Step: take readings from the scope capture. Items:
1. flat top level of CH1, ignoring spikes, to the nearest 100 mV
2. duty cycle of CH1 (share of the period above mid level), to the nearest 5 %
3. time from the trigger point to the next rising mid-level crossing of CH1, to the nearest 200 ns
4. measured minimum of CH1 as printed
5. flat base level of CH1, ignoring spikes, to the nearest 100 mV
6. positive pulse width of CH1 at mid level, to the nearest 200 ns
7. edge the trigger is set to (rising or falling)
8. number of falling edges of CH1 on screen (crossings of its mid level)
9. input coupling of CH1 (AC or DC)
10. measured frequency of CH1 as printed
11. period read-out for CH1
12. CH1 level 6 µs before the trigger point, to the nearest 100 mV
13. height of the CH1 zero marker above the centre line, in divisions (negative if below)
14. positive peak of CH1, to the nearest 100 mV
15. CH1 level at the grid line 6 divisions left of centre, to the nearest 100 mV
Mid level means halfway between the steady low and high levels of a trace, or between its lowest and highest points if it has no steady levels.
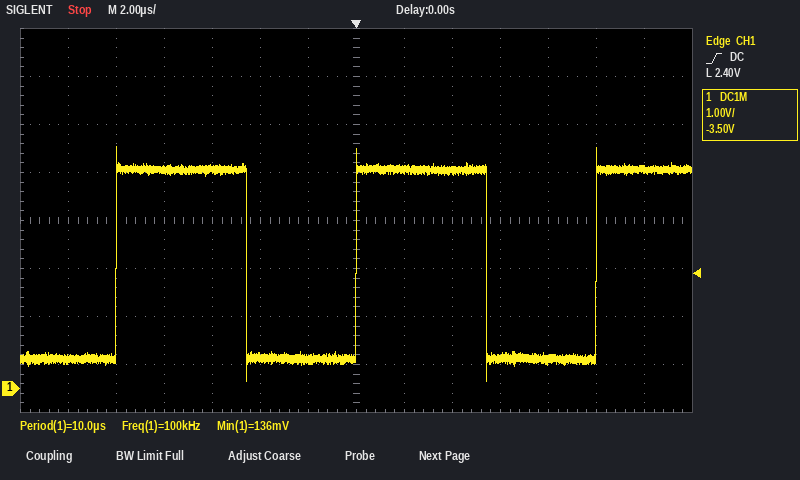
4.6 V
55 %
10.0 µs
136 mV
600 mV
5.4 µs
rising
2
DC
100 kHz
10.0 µs
4.6 V
-3.5 div
5.0 V
600 mV
